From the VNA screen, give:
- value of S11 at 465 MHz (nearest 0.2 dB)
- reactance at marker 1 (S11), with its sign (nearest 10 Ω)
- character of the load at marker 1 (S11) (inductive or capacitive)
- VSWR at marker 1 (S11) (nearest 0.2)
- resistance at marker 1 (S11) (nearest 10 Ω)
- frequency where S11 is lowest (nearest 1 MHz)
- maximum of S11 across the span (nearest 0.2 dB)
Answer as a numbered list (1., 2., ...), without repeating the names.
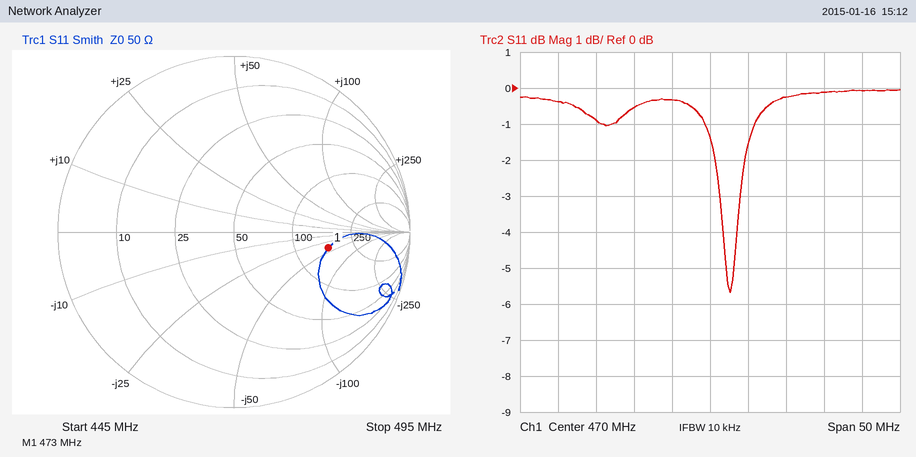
1. -0.4 dB
2. -40 Ω
3. capacitive
4. 3.4
5. 160 Ω
6. 473 MHz
7. 0.0 dB
